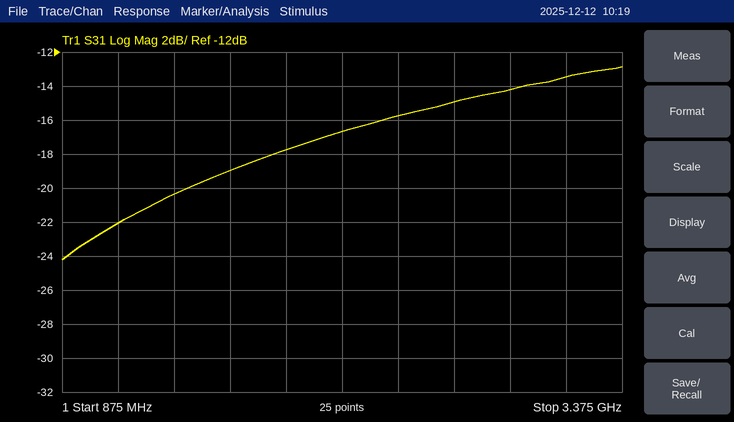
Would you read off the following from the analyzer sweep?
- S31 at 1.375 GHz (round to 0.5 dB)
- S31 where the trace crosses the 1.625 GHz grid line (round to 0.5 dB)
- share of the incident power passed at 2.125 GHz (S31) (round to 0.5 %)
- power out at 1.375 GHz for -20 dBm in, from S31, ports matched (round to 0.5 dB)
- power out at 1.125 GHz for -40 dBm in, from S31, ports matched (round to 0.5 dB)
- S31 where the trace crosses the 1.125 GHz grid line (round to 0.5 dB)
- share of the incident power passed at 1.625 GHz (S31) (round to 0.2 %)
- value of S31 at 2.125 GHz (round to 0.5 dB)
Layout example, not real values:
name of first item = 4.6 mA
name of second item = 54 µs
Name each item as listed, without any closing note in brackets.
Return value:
S31 at 1.375 GHz = -20.5 dB
S31 where the trace crosses the 1.625 GHz grid line = -19.0 dB
share of the incident power passed at 2.125 GHz (S31) = 2.0 %
power out at 1.375 GHz for -20 dBm in, from S31, ports matched = -40.5 dBm
power out at 1.125 GHz for -40 dBm in, from S31, ports matched = -62.0 dBm
S31 where the trace crosses the 1.125 GHz grid line = -22.0 dB
share of the incident power passed at 1.625 GHz (S31) = 1.2 %
value of S31 at 2.125 GHz = -16.5 dB
